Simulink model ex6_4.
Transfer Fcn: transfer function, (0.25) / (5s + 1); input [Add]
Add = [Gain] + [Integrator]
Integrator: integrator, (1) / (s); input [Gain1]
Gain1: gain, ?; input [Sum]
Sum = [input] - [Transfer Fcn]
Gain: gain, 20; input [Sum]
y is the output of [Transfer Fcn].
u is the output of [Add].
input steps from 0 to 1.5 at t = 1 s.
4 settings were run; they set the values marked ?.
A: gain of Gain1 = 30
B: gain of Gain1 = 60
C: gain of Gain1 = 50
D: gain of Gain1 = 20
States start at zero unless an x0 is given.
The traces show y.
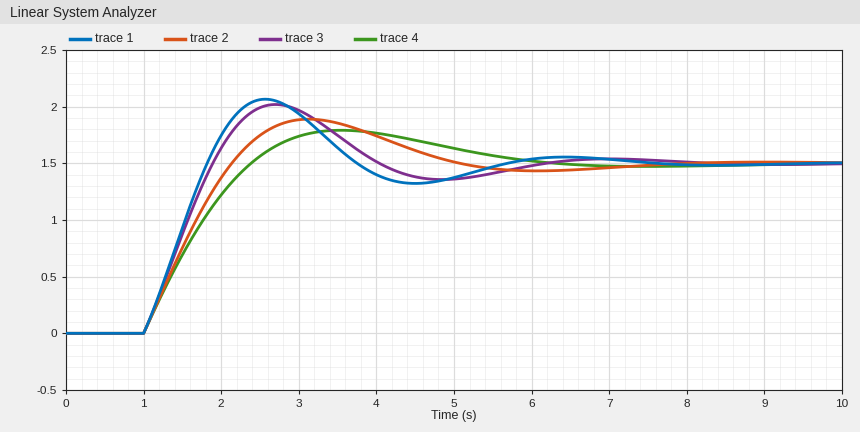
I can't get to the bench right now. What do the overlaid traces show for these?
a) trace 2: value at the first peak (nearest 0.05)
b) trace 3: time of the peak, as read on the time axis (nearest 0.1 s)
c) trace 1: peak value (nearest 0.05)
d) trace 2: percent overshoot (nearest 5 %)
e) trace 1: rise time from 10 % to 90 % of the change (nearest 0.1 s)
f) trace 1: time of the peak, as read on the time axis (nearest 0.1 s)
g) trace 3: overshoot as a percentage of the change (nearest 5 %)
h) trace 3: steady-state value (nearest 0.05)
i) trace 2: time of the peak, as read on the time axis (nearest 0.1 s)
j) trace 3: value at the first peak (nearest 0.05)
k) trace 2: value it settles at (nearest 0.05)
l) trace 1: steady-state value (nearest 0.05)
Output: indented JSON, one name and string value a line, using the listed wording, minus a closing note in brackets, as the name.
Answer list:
{
  "trace 2: value at the first peak": "1.90",
  "trace 3: time of the peak, as read on the time axis": "2.7 s",
  "trace 1: peak value": "2.05",
  "trace 2: percent overshoot": "25 %",
  "trace 1: rise time from 10 % to 90 % of the change": "0.6 s",
  "trace 1: time of the peak, as read on the time axis": "2.6 s",
  "trace 3: overshoot as a percentage of the change": "35 %",
  "trace 3: steady-state value": "1.50",
  "trace 2: time of the peak, as read on the time axis": "3.1 s",
  "trace 3: value at the first peak": "2.00",
  "trace 2: value it settles at": "1.50",
  "trace 1: steady-state value": "1.50"
}
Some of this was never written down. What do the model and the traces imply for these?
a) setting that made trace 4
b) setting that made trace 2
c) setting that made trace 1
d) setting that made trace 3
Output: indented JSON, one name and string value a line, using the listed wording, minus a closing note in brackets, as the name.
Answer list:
{
  "setting that made trace 4": "D",
  "setting that made trace 2": "A",
  "setting that made trace 1": "B",
  "setting that made trace 3": "C"
}
